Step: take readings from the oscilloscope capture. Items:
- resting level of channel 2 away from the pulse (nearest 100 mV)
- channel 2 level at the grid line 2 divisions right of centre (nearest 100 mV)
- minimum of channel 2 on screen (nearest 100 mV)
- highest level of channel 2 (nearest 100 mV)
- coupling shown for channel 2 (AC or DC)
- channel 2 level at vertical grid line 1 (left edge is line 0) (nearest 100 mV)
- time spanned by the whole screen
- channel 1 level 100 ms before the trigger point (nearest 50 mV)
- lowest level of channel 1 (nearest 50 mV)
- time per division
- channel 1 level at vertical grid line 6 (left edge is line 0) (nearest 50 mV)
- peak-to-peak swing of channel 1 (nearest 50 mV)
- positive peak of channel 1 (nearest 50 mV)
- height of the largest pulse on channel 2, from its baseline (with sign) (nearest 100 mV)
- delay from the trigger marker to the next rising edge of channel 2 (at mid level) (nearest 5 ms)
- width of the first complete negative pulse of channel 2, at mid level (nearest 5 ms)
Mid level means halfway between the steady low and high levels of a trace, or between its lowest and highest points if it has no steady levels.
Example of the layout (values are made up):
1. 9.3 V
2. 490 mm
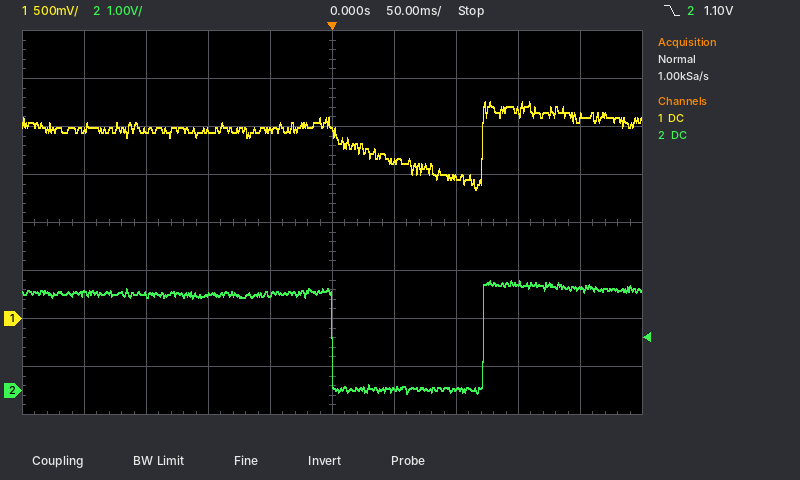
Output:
1. 2.0 V
2. 0.0 V
3. -100 mV
4. 2.3 V
5. DC
6. 2.0 V
7. 500 ms
8. 1.95 V
9. 1.35 V
10. 50 ms
11. 1.65 V
12. 900 mV
13. 2.25 V
14. -2.1 V
15. 120 ms
16. 120 ms
